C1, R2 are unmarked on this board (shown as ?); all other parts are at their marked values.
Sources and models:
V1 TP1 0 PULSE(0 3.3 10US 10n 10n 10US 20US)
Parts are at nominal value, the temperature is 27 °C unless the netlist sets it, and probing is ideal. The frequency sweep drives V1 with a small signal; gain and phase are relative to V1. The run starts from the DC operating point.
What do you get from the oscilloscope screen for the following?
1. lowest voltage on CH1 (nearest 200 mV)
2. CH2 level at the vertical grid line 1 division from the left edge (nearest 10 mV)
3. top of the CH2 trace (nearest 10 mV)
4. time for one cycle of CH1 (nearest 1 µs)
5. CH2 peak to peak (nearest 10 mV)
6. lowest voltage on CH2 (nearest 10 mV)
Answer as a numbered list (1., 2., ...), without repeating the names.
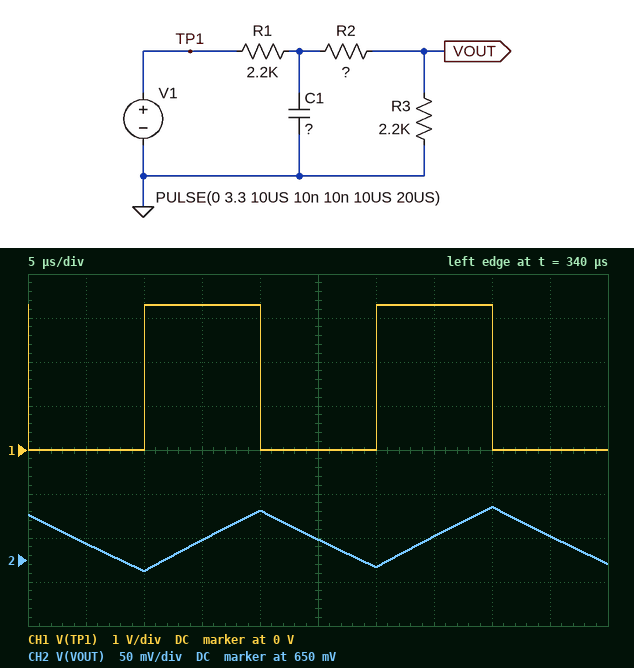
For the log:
1. 0 V
2. 670 mV
3. 710 mV
4. 20 µs
5. 70 mV
6. 640 mV
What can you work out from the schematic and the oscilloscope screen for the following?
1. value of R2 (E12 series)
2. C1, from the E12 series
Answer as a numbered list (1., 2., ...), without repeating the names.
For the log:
1. 820 Ω
2. 82 nF
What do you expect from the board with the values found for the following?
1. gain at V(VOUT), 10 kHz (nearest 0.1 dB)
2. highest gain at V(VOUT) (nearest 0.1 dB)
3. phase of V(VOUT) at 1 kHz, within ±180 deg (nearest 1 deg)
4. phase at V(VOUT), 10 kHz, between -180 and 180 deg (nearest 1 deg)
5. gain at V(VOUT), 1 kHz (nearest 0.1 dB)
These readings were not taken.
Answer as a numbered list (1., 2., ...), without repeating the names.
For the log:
1. -23.9 dB
2. -7.5 dB
3. -33 deg
4. -81 deg
5. -9.1 dB
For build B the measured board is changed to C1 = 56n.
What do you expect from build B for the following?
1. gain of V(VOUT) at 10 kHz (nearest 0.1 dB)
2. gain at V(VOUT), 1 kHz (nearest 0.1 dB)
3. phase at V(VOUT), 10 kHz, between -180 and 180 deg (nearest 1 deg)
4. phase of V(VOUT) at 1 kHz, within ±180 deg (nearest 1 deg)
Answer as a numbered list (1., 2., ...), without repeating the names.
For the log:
1. -20.7 dB
2. -8.3 dB
3. -77 deg
4. -24 deg
